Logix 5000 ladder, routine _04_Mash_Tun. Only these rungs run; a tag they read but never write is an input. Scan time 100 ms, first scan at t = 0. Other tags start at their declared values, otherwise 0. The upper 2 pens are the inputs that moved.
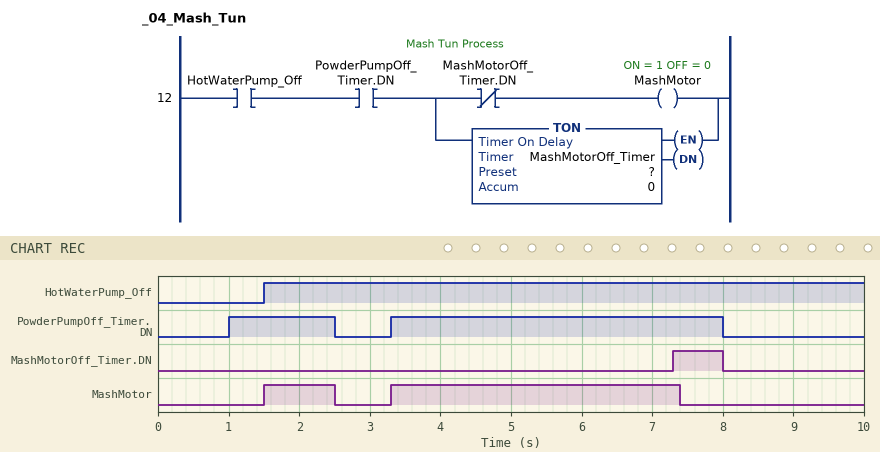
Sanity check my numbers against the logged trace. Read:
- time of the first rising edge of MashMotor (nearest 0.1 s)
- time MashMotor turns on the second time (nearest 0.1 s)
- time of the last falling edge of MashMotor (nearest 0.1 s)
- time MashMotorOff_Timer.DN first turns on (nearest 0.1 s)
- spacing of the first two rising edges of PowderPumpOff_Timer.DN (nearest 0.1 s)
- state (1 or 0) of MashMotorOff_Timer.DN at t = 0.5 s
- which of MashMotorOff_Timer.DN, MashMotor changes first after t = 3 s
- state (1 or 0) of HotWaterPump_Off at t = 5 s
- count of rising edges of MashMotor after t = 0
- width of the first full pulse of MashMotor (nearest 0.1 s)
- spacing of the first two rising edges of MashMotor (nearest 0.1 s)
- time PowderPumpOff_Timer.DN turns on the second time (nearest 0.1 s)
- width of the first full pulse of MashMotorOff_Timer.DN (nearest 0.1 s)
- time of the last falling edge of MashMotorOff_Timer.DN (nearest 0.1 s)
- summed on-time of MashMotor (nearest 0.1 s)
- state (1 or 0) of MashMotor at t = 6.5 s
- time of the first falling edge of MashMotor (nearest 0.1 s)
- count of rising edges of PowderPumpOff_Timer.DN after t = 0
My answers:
1.5 s
3.3 s
7.4 s
7.3 s
2.3 s
0
MashMotor
1
2
1.0 s
1.8 s
3.3 s
0.7 s
8.0 s
5.1 s
1
2.5 s
2
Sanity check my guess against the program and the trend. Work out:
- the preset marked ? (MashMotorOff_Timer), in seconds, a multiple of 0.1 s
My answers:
4.0 s
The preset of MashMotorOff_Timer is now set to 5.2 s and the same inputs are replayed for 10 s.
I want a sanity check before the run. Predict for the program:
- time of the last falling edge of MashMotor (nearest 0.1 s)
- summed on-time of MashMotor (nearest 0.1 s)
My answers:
8.0 s
5.7 s
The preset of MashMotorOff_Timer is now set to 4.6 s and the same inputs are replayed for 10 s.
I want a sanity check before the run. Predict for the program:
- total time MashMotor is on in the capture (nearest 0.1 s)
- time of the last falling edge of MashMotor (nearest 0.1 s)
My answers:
5.7 s
8.0 s
